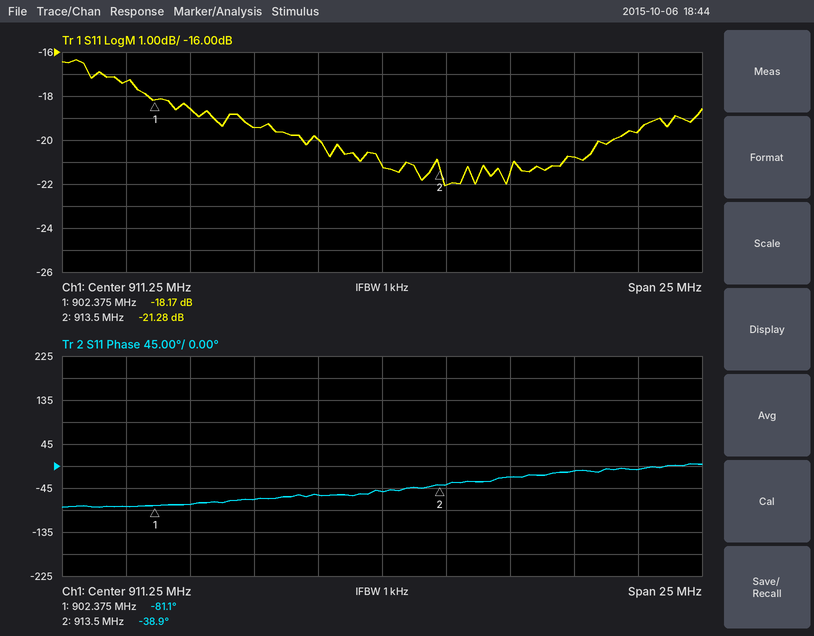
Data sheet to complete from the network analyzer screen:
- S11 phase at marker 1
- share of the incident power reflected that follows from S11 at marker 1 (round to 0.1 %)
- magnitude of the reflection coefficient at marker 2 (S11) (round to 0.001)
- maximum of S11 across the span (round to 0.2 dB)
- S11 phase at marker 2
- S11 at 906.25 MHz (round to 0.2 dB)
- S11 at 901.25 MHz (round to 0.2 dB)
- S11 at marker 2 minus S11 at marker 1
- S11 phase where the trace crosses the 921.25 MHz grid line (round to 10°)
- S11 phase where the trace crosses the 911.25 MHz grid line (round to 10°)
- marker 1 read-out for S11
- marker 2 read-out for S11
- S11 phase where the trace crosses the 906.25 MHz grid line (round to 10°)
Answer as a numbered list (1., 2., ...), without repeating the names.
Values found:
1. -81.1°
2. 1.5 %
3. 0.086
4. -16.4 dB
5. -38.9°
6. -19.4 dB
7. -17.4 dB
8. -3.11 dB
9. -10°
10. -50°
11. -18.17 dB
12. -21.28 dB
13. -70°
